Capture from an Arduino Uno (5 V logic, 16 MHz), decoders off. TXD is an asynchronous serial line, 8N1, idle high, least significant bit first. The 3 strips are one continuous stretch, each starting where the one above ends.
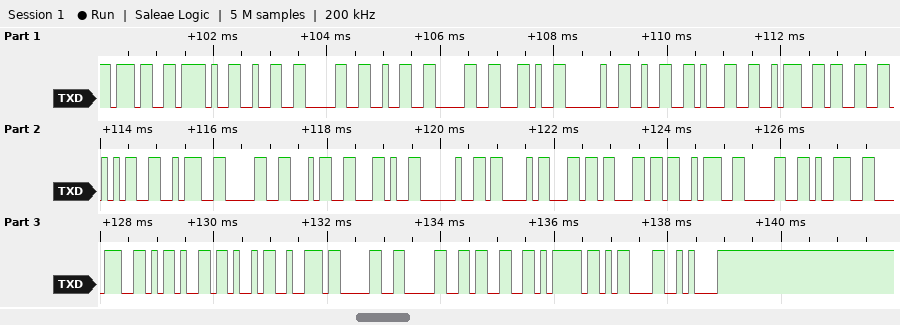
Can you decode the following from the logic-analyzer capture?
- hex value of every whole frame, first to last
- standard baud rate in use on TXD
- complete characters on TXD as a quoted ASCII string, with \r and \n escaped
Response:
0x37 0x2F 0x32 0x30 0x32 0x30 0x2C 0x20 0x32 0x31 0x3A 0x33 0x35 0x3A 0x30 0x34 0x2C 0x20 0x43 0x6C 0x6C 0x3A 0x30 0x39 0x38 0x2D 0x4B 0x72 0x30 0x30 0x33 0x7D 0x0D 0x0A
9600 baud
"7/2020, 21:35:04, Cll:098-Kr003}\r\n"
